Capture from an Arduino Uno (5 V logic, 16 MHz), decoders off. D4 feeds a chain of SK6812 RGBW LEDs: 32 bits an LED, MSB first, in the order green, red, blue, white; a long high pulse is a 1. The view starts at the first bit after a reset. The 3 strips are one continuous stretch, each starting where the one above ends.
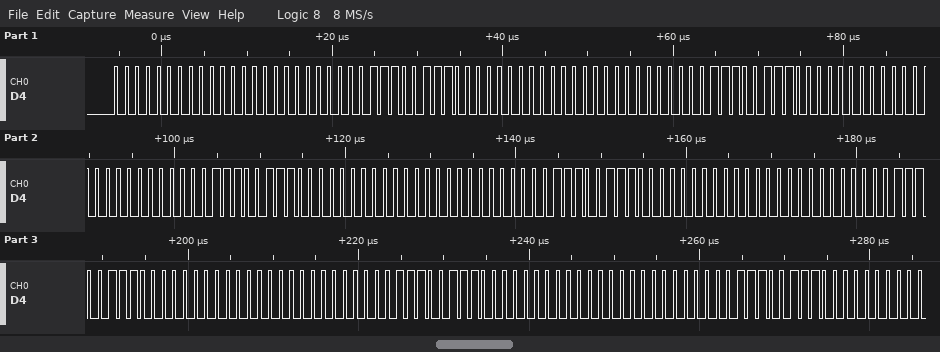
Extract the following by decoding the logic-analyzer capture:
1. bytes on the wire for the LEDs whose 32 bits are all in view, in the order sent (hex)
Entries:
00 00 00 E7 00 00 00 E7 00 00 00 E7 00 00 00 E7 00 00 00 E7 00 00 00 E7 00 00 00 E7
